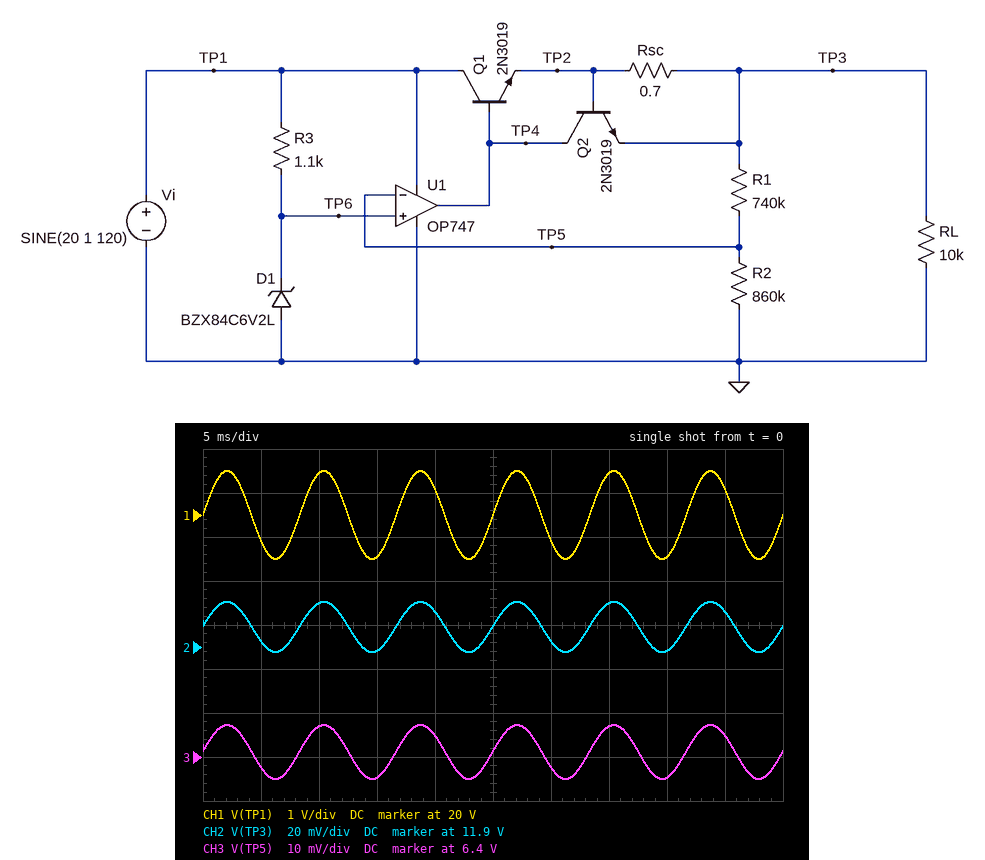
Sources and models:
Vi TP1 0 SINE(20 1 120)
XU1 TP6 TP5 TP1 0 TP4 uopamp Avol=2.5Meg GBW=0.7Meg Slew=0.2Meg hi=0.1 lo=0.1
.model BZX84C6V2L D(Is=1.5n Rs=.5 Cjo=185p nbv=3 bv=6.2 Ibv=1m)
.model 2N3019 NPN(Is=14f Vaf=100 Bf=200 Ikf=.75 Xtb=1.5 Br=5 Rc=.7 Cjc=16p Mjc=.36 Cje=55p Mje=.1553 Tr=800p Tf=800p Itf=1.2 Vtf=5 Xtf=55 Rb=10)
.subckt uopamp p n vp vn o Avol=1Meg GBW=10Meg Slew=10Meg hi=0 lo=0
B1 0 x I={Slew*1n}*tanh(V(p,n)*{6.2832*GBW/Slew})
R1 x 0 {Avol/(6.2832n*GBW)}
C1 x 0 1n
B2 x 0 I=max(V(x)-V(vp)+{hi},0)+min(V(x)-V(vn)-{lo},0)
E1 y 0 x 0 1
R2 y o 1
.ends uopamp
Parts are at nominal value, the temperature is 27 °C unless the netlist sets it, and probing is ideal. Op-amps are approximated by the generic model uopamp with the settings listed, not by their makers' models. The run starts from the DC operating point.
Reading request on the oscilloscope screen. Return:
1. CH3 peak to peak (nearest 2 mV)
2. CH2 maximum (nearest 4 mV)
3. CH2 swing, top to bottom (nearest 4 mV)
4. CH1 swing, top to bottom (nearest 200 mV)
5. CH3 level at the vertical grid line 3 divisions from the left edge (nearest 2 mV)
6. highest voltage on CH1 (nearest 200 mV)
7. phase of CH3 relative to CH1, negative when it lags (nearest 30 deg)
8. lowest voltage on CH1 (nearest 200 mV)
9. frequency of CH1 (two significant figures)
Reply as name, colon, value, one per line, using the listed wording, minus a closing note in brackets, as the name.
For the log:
CH3 peak to peak: 12 mV
CH2 maximum: 11.920 V
CH2 swing, top to bottom: 24 mV
CH1 swing, top to bottom: 2.0 V
CH3 level at the vertical grid line 3 divisions from the left edge: 6.396 V
highest voltage on CH1: 21.0 V
phase of CH3 relative to CH1, negative when it lags: 0 deg
lowest voltage on CH1: 19.0 V
frequency of CH1: 120 Hz
